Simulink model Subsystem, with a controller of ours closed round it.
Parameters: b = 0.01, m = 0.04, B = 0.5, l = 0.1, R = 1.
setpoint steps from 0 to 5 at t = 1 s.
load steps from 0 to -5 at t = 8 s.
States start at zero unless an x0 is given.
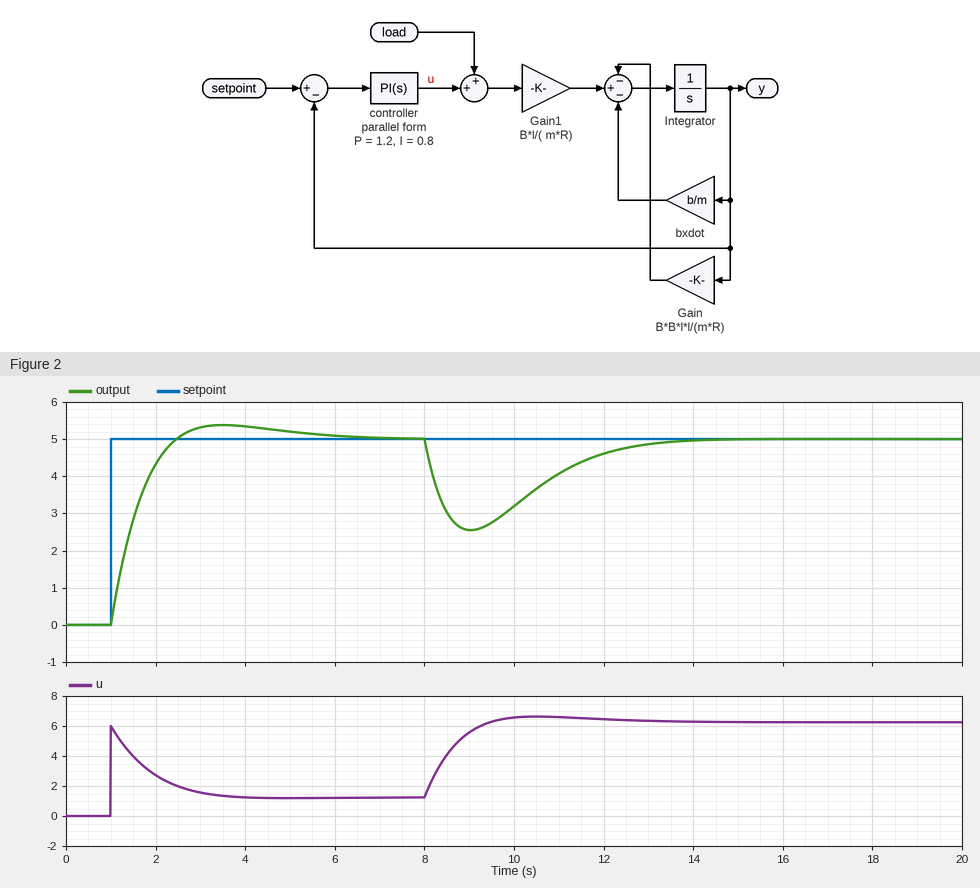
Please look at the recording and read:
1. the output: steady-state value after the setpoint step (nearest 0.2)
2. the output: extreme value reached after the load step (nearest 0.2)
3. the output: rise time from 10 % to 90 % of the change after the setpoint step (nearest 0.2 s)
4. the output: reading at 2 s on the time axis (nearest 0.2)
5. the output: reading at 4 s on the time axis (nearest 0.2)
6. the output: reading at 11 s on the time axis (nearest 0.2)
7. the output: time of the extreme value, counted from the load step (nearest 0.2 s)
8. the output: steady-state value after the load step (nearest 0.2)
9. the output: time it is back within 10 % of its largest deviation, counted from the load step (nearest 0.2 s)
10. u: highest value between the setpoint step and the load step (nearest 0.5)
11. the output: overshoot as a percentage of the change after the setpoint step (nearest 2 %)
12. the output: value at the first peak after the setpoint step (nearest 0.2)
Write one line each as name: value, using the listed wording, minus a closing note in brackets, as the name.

the output: steady-state value after the setpoint step: 5.0
the output: extreme value reached after the load step: 2.6
the output: rise time from 10 % to 90 % of the change after the setpoint step: 1.0 s
the output: reading at 2 s on the time axis: 4.4
the output: reading at 4 s on the time axis: 5.4
the output: reading at 11 s on the time axis: 4.0
the output: time of the extreme value, counted from the load step: 1.0 s
the output: steady-state value after the load step: 5.0
the output: time it is back within 10 % of its largest deviation, counted from the load step: 4.4 s
u: highest value between the setpoint step and the load step: 6.0
the output: overshoot as a percentage of the change after the setpoint step: 8 %
the output: value at the first peak after the setpoint step: 5.4
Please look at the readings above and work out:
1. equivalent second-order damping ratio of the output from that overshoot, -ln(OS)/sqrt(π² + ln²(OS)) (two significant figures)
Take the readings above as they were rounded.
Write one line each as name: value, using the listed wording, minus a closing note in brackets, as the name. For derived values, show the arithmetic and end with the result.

equivalent second-order damping ratio of the output from that overshoot, -ln(OS)/sqrt(π² + ln²(OS)): ln(0.08) = -2.526; 2.526 / sqrt(9.870 + 6.379) = 0.63
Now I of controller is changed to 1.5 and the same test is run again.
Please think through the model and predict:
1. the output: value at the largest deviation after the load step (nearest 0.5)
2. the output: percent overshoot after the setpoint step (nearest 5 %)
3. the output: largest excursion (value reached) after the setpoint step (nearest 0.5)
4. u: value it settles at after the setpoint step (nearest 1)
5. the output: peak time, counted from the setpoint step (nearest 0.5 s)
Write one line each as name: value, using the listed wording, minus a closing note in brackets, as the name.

the output: value at the largest deviation after the load step: 3.0
the output: percent overshoot after the setpoint step: 15 %
the output: largest excursion (value reached) after the setpoint step: 6.0
u: value it settles at after the setpoint step: 1
the output: peak time, counted from the setpoint step: 2.0 s
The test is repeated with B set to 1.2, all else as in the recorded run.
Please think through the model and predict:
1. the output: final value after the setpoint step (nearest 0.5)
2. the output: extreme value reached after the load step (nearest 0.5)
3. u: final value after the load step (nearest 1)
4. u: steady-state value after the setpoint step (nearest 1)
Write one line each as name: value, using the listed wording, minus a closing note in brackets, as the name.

the output: final value after the setpoint step: 5.0
the output: extreme value reached after the load step: 2.0
u: final value after the load step: 6
u: steady-state value after the setpoint step: 1
